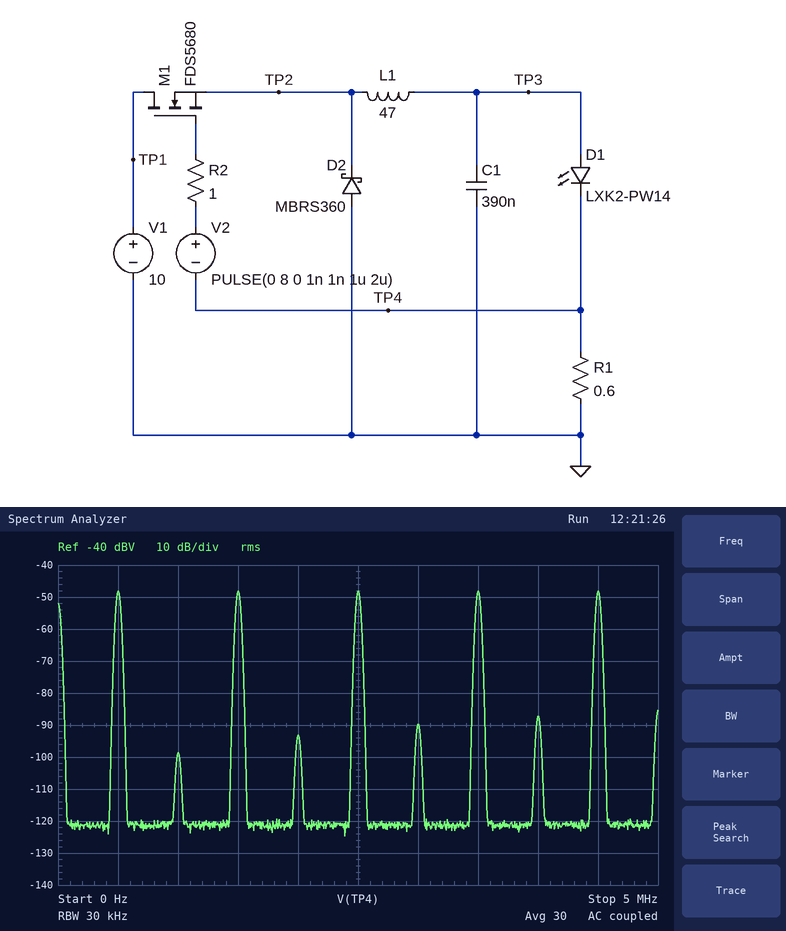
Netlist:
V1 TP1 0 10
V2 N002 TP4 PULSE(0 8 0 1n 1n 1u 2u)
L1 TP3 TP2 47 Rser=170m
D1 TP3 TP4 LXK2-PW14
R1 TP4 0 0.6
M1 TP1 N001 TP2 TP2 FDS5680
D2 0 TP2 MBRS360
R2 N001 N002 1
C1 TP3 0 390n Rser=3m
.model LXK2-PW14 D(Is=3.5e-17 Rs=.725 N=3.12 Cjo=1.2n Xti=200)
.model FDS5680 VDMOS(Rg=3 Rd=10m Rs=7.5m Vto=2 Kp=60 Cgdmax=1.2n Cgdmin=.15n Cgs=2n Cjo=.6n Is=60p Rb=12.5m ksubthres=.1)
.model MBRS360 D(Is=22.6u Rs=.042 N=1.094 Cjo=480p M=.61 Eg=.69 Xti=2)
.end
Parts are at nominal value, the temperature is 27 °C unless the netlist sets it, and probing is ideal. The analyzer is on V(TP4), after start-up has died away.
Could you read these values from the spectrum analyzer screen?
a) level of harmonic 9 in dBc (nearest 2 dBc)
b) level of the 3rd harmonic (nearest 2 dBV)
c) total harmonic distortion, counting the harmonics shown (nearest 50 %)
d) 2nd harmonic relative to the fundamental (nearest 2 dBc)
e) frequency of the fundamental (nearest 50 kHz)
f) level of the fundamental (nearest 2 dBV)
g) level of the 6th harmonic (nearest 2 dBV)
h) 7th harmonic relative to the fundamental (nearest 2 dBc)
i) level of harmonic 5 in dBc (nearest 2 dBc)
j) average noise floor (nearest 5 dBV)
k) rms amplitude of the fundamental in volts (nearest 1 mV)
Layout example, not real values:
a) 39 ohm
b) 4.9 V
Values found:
a) 0 dBc
b) -48 dBV
c) 200 %
d) -50 dBc
e) 500 kHz
f) -48 dBV
g) -90 dBV
h) 0 dBc
i) 0 dBc
j) -120 dBV
k) 4 mV
